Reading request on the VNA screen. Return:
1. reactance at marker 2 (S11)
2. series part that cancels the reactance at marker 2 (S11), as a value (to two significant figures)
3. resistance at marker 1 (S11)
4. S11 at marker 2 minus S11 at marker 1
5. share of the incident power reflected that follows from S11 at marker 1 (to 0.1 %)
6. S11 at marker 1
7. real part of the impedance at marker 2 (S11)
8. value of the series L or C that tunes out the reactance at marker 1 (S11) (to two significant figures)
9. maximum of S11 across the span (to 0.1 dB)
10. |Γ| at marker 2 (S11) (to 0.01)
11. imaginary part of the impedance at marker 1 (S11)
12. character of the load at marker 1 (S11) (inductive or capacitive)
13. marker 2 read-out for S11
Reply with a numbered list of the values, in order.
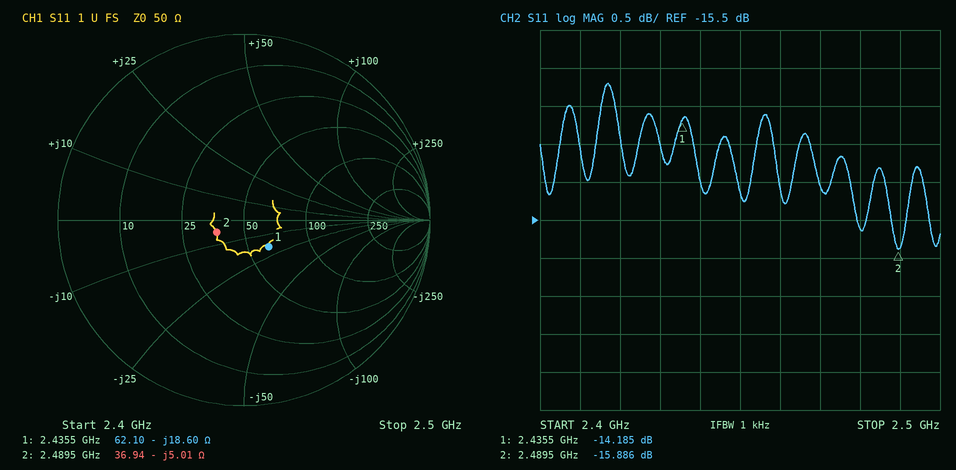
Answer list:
1. -5.01 Ω
2. 320 pH
3. 62.10 Ω
4. -1.701 dB
5. 3.8 %
6. -14.185 dB
7. 36.94 Ω
8. 1.2 nH
9. -13.7 dB
10. 0.16
11. -18.60 Ω
12. capacitive
13. -15.886 dB
